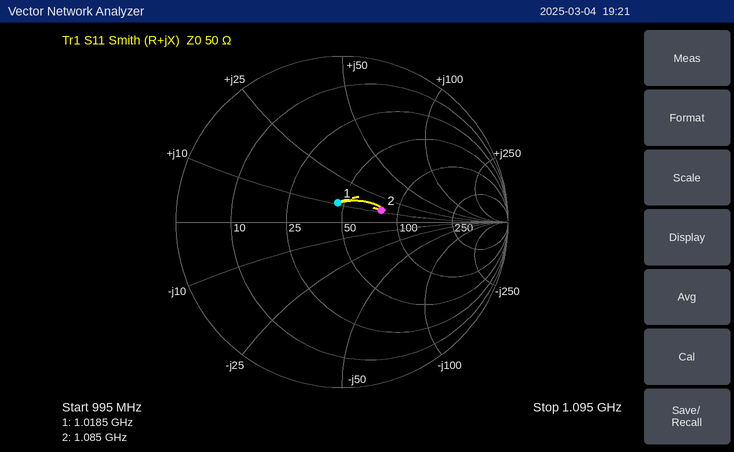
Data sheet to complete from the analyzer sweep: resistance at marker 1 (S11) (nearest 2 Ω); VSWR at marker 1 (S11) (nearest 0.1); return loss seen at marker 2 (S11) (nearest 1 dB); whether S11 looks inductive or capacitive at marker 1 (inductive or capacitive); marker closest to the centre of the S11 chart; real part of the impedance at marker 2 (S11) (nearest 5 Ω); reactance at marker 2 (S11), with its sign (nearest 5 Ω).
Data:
46 Ω
1.3
12 dB
inductive
marker 1
80 Ω
+10 Ω
